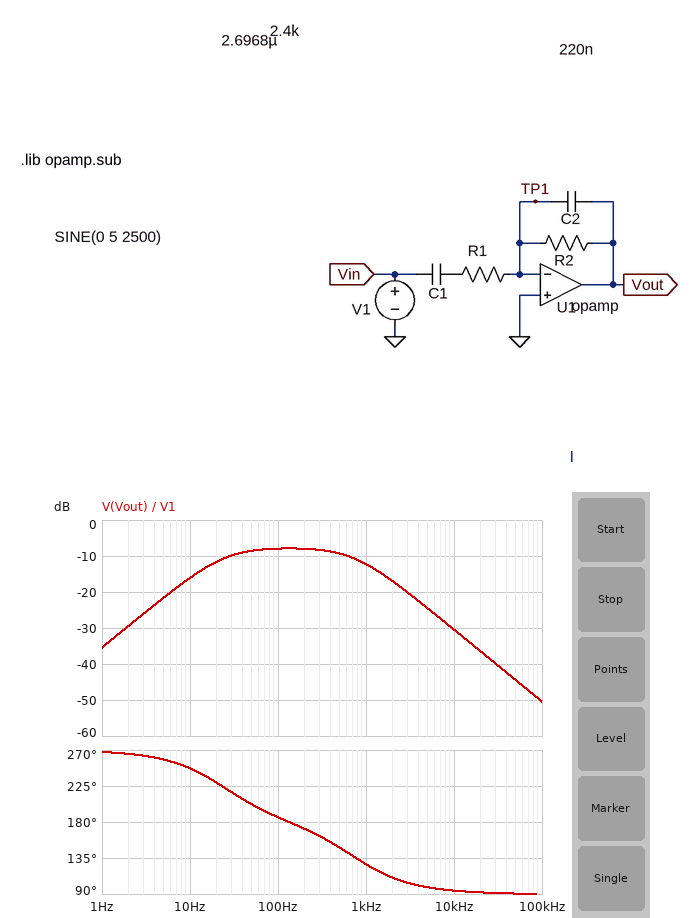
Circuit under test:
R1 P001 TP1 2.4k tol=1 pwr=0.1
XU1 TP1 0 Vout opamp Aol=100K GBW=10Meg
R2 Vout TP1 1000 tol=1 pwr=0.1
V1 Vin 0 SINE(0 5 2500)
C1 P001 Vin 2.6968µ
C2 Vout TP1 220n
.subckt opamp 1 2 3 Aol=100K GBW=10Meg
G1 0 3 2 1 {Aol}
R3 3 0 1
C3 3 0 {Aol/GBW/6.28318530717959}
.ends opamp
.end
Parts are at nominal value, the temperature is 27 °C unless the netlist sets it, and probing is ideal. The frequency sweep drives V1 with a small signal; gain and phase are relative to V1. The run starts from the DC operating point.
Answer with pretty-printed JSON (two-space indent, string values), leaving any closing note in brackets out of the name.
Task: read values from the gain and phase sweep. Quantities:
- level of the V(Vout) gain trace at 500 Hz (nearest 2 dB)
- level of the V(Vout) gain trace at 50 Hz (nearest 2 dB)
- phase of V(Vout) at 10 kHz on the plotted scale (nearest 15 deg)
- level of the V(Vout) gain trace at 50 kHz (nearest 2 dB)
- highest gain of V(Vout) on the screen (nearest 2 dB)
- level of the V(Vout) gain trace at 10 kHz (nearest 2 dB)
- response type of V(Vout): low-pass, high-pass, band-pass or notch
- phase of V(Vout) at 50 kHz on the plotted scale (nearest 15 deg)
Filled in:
{
  "level of the V(Vout) gain trace at 500 Hz": "-10 dB",
  "level of the V(Vout) gain trace at 50 Hz": "-8 dB",
  "phase of V(Vout) at 10 kHz on the plotted scale": "90 deg",
  "level of the V(Vout) gain trace at 50 kHz": "-44 dB",
  "highest gain of V(Vout) on the screen": "-8 dB",
  "level of the V(Vout) gain trace at 10 kHz": "-30 dB",
  "response type of V(Vout): low-pass, high-pass, band-pass or notch": "band-pass",
  "phase of V(Vout) at 50 kHz on the plotted scale": "90 deg"
}
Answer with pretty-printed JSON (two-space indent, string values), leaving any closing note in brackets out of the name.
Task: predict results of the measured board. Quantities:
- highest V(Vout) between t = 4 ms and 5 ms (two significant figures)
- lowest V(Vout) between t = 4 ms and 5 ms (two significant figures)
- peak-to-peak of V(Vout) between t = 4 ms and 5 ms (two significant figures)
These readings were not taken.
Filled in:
{
  "highest V(Vout) between t = 4 ms and 5 ms": "590 mV",
  "lowest V(Vout) between t = 4 ms and 5 ms": "-570 mV",
  "peak-to-peak of V(Vout) between t = 4 ms and 5 ms": "1.2 V"
}
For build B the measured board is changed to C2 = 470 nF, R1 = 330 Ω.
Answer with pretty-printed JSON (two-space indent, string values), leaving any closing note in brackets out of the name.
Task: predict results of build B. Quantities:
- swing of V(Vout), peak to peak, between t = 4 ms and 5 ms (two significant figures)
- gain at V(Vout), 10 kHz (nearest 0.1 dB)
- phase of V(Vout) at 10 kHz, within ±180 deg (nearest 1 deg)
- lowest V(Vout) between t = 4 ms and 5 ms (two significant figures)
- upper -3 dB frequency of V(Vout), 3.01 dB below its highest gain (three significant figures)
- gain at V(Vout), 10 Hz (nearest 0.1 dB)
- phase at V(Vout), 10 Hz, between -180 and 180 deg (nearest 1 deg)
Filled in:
{
  "swing of V(Vout), peak to peak, between t = 4 ms and 5 ms": "4.1 V",
  "gain at V(Vout), 10 kHz": "-19.8 dB",
  "phase of V(Vout) at 10 kHz, within ±180 deg": "93 deg",
  "lowest V(Vout) between t = 4 ms and 5 ms": "-2.0 V",
  "upper -3 dB frequency of V(Vout), 3.01 dB below its highest gain": "616 Hz",
  "gain at V(Vout), 10 Hz": "-15.4 dB",
  "phase at V(Vout), 10 Hz, between -180 and 180 deg": "-95 deg"
}
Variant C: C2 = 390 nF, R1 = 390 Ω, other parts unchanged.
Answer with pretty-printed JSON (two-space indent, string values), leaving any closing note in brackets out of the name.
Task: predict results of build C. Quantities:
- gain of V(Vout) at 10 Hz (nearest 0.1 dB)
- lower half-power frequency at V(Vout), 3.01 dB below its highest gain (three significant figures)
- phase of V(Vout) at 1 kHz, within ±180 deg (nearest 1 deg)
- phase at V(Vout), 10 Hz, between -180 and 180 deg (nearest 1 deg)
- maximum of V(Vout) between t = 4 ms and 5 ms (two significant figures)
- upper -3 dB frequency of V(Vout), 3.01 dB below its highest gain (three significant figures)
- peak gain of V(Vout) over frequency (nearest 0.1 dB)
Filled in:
{
  "gain of V(Vout) at 10 Hz": "-15.4 dB",
  "lower half-power frequency at V(Vout), 3.01 dB below its highest gain": "94.4 Hz",
  "phase of V(Vout) at 1 kHz, within ±180 deg": "121 deg",
  "phase at V(Vout), 10 Hz, between -180 and 180 deg": "-95 deg",
  "maximum of V(Vout) between t = 4 ms and 5 ms": "2.1 V",
  "upper -3 dB frequency of V(Vout), 3.01 dB below its highest gain": "654 Hz",
  "peak gain of V(Vout) over frequency": "5.4 dB"
}
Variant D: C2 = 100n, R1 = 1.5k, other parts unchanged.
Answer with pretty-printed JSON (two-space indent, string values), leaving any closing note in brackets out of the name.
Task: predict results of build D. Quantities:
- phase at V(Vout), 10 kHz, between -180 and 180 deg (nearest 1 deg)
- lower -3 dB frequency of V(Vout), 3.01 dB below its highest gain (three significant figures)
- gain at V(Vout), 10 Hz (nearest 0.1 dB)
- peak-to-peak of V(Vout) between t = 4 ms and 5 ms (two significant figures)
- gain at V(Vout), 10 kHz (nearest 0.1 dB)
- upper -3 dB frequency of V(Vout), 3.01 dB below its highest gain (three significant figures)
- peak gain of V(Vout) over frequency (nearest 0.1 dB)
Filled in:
{
  "phase at V(Vout), 10 kHz, between -180 and 180 deg": "99 deg",
  "lower -3 dB frequency of V(Vout), 3.01 dB below its highest gain": "37.5 Hz",
  "gain at V(Vout), 10 Hz": "-15.7 dB",
  "peak-to-peak of V(Vout) between t = 4 ms and 5 ms": "3.6 V",
  "gain at V(Vout), 10 kHz": "-19.6 dB",
  "upper -3 dB frequency of V(Vout), 3.01 dB below its highest gain": "1.67 kHz",
  "peak gain of V(Vout) over frequency": "-3.7 dB"
}
